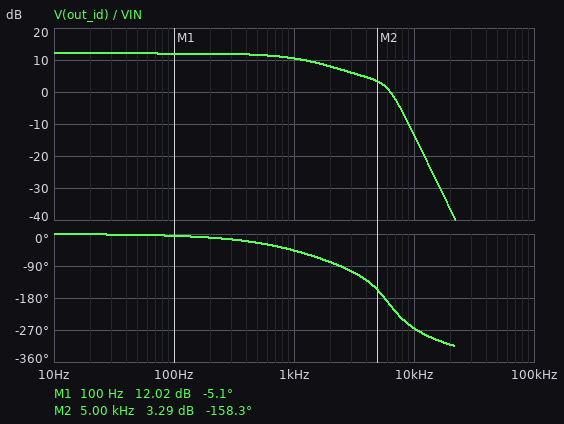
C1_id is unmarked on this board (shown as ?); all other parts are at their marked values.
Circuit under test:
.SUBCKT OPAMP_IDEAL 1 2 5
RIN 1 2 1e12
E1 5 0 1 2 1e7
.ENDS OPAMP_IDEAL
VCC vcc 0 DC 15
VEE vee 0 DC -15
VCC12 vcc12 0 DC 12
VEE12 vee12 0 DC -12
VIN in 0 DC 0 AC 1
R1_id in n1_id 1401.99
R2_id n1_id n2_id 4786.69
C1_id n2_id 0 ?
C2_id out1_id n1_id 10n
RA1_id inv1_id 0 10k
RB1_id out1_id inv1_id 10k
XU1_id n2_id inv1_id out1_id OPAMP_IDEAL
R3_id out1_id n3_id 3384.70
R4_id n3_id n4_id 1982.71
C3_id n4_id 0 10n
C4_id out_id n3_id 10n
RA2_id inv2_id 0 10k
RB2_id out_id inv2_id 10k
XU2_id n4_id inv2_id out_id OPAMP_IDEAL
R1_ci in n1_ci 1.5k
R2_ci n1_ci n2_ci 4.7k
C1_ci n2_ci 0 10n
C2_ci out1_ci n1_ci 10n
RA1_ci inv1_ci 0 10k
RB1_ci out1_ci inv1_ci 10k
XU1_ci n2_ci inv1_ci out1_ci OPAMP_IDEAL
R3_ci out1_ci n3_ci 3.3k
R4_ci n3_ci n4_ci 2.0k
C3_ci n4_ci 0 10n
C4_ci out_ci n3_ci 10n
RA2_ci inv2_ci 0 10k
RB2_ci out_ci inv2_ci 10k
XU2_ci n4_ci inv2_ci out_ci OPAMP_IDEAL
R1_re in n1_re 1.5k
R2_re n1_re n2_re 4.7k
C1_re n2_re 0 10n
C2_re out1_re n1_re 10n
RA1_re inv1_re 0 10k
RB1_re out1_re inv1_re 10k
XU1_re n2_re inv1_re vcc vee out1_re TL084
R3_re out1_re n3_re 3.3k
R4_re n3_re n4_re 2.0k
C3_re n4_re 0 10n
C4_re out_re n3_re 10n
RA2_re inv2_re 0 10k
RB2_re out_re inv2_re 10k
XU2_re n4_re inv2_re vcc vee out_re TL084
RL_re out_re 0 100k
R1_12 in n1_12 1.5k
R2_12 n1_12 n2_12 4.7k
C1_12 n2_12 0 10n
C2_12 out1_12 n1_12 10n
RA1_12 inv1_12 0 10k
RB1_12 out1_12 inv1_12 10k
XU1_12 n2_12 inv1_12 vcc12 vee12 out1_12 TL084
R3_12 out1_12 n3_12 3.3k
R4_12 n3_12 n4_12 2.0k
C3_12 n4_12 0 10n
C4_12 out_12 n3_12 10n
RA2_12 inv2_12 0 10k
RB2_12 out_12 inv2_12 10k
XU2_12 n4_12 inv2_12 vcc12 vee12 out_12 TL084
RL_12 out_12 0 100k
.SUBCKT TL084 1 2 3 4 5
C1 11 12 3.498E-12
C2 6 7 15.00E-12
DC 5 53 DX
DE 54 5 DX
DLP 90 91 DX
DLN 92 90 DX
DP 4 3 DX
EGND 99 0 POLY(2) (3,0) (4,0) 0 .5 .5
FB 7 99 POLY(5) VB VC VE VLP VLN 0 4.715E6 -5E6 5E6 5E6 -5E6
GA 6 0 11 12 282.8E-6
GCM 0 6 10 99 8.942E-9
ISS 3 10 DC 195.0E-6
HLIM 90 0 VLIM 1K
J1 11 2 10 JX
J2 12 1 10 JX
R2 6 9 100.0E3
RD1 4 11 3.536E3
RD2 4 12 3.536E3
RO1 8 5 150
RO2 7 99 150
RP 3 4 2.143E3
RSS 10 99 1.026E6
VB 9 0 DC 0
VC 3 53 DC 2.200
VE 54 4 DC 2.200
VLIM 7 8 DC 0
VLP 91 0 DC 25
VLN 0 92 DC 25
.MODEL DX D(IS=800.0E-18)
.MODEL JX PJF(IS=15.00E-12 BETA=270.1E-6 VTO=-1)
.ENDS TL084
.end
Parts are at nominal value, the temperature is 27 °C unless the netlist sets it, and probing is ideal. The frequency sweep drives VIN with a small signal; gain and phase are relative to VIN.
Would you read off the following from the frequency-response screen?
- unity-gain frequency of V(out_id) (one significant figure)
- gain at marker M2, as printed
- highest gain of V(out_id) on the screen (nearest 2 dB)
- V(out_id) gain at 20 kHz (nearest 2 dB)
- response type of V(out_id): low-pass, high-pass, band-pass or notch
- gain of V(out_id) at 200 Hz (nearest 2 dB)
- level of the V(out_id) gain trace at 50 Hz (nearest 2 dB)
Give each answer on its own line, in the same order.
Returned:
6 kHz
3.29 dB
12 dB
-36 dB
low-pass
12 dB
12 dB
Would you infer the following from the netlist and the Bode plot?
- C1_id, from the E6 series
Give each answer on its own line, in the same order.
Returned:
22 nF
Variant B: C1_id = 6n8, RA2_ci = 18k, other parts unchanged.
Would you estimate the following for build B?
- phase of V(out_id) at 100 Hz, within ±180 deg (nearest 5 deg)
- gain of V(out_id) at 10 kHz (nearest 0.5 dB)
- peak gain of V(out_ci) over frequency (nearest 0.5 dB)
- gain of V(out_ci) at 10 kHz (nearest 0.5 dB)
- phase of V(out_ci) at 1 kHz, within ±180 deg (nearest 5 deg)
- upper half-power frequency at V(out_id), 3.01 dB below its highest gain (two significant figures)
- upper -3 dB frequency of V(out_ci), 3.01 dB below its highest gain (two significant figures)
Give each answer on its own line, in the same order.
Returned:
0 deg
0 dB
10.0 dB
-9.5 dB
-30 deg
6.7 kHz
4.2 kHz
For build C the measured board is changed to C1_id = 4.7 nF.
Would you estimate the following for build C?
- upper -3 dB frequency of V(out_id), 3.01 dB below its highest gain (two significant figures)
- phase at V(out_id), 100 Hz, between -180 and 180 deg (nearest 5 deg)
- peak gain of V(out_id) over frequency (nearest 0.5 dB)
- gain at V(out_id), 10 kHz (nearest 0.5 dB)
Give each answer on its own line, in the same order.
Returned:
7.5 kHz
0 deg
17.0 dB
6.0 dB
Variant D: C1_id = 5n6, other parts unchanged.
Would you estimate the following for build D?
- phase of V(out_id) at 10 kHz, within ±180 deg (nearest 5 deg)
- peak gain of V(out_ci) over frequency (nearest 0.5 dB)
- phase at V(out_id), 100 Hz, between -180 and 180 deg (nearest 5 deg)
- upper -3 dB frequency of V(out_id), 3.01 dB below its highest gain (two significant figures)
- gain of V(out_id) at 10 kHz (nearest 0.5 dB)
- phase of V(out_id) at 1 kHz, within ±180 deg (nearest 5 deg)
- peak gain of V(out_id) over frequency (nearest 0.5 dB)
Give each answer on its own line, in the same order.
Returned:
105 deg
12.0 dB
0 deg
7.1 kHz
3.0 dB
-15 deg
16.0 dB
